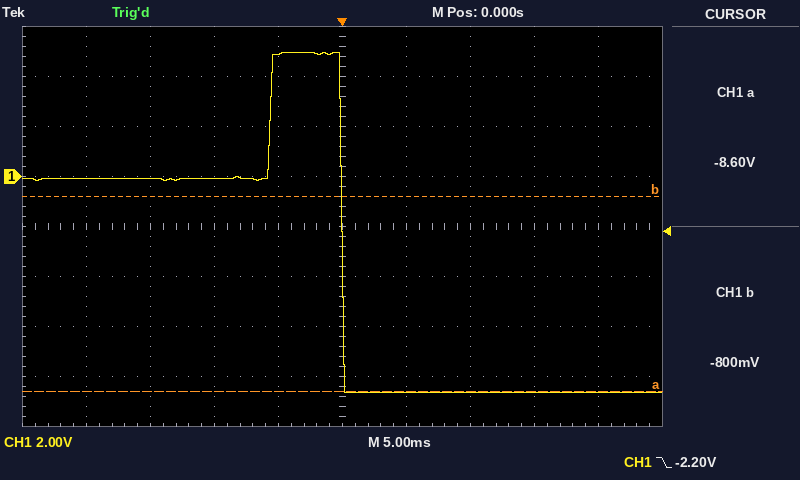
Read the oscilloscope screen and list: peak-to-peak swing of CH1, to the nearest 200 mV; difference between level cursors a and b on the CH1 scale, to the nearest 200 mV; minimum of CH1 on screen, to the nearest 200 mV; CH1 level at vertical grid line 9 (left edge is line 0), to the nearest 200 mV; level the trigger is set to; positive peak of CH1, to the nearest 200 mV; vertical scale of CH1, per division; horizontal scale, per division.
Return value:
13.6 V
7.8 V
-8.6 V
-8.6 V
-2.20 V
5.0 V
2 V
5 ms
